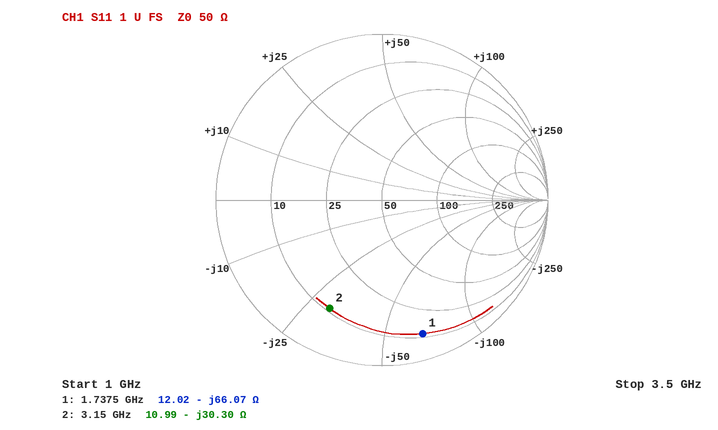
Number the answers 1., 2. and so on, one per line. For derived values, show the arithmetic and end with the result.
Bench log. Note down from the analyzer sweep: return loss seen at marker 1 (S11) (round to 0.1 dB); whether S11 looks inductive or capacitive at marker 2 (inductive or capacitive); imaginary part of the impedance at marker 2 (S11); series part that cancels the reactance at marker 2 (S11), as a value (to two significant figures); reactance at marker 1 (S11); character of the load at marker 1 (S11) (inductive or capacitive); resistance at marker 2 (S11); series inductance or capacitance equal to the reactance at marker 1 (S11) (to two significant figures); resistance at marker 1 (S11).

1. 1.5 dB
2. capacitive
3. -30.30 Ω
4. L = 30.3 Ω/(2π × 3.15 GHz) ≈ 1.5 nH
5. -66.07 Ω
6. capacitive
7. 10.99 Ω
8. C = 1/(2π × 1.7375 GHz × 66.07 Ω) ≈ 1.4 pF
9. 12.02 Ω
